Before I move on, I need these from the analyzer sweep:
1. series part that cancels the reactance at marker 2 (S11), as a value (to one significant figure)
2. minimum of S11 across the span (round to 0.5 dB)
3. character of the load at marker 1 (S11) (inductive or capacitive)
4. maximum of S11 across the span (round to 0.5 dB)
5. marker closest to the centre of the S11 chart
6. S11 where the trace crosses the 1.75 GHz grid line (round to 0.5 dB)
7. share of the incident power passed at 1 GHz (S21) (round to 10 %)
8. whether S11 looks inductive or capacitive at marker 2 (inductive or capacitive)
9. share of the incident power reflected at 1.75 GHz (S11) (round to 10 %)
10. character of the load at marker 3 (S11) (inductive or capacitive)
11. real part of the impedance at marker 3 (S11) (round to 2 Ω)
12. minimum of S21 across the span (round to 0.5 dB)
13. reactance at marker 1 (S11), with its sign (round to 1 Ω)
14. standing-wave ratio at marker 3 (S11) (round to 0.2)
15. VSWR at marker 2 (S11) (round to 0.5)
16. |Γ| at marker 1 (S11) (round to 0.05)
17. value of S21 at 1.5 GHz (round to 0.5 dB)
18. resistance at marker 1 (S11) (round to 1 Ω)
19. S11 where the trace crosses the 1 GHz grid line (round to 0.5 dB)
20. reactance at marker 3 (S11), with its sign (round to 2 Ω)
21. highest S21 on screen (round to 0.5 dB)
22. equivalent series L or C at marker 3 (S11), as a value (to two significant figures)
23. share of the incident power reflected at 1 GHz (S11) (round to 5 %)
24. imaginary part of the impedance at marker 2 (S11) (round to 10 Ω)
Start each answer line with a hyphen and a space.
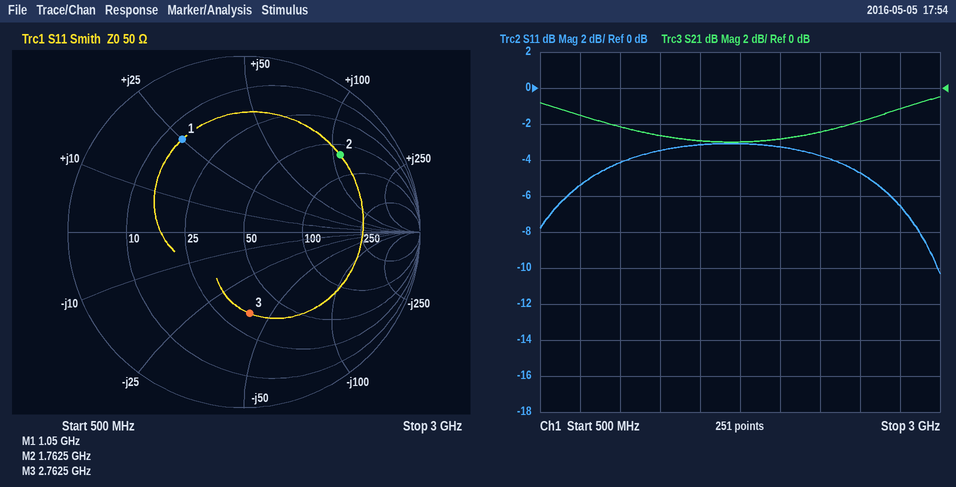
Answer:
- 800 fF
- -10.5 dB
- inductive
- -3.0 dB
- marker 3
- -3.0 dB
- 60 %
- inductive
- 50 %
- capacitive
- 34 Ω
- -3.0 dB
- +25 Ω
- 2.8
- 5.5
- 0.65
- -3.0 dB
- 14 Ω
- -4.0 dB
- -40 Ω
- -0.5 dB
- 1.4 pF
- 40 %
- +110 Ω
